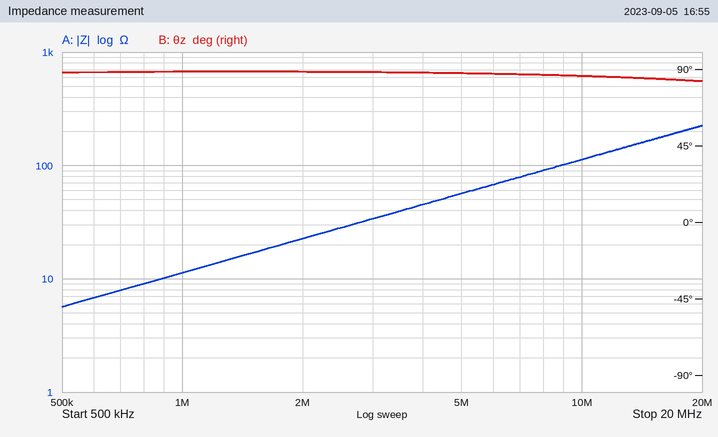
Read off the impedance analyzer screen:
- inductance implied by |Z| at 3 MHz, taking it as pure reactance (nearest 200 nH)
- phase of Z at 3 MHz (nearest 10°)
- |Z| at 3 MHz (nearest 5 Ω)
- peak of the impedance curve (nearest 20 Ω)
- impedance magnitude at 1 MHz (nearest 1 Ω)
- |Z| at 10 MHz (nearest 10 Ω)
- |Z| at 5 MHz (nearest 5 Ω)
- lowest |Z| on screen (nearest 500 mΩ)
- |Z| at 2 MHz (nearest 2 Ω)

1.8 µH
90°
35 Ω
220 Ω
11 Ω
110 Ω
55 Ω
5.5 Ω
22 Ω
